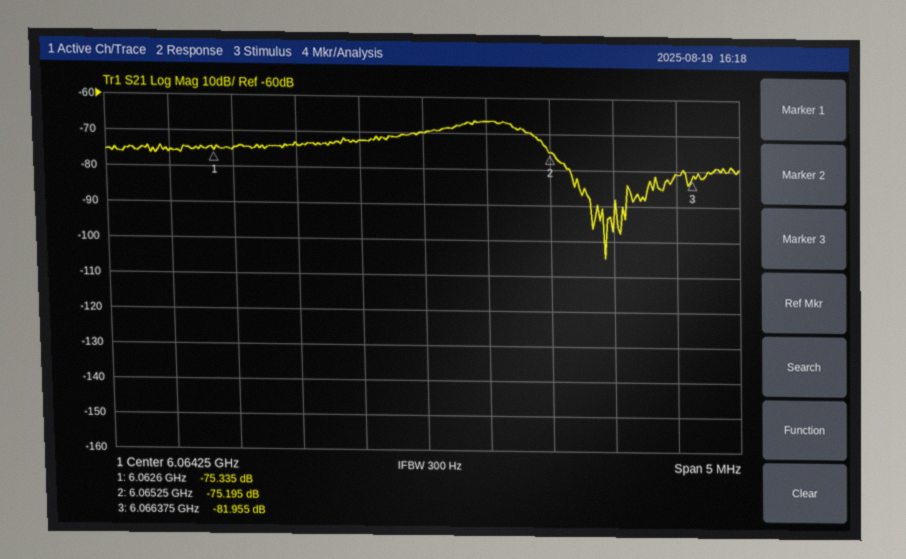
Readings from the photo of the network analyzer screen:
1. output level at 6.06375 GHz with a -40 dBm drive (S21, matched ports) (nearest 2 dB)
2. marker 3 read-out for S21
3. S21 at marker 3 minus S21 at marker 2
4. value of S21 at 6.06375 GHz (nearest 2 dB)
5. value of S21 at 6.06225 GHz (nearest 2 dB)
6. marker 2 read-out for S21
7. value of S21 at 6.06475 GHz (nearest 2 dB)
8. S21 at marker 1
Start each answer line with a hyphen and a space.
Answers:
- -112 dBm
- -81.955 dB
- -6.760 dB
- -72 dB
- -76 dB
- -75.195 dB
- -66 dB
- -75.335 dB
